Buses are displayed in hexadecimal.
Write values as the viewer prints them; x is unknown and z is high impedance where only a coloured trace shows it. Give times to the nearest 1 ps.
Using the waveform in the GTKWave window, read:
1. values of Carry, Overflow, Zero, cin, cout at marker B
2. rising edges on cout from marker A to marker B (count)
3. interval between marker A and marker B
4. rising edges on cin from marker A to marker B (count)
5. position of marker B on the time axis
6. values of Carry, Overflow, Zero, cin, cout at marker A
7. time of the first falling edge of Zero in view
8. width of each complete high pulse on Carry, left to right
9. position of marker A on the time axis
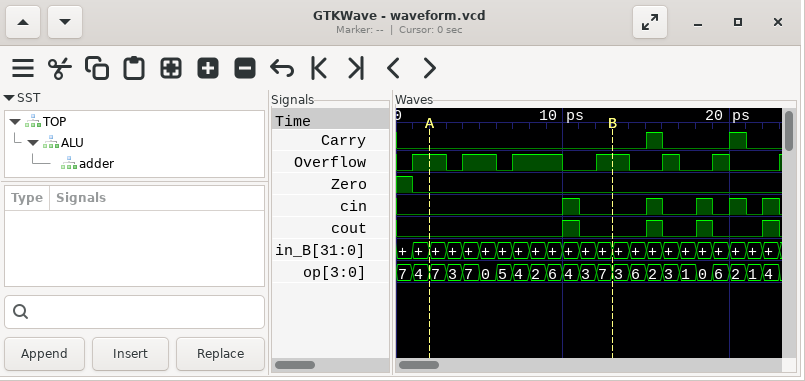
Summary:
Carry=0, Overflow=1, Zero=0, cin=0, cout=0
1
11 ps
1
13 ps
Carry=0, Overflow=1, Zero=0, cin=0, cout=0
1 ps
1 ps, 1 ps
2 ps
